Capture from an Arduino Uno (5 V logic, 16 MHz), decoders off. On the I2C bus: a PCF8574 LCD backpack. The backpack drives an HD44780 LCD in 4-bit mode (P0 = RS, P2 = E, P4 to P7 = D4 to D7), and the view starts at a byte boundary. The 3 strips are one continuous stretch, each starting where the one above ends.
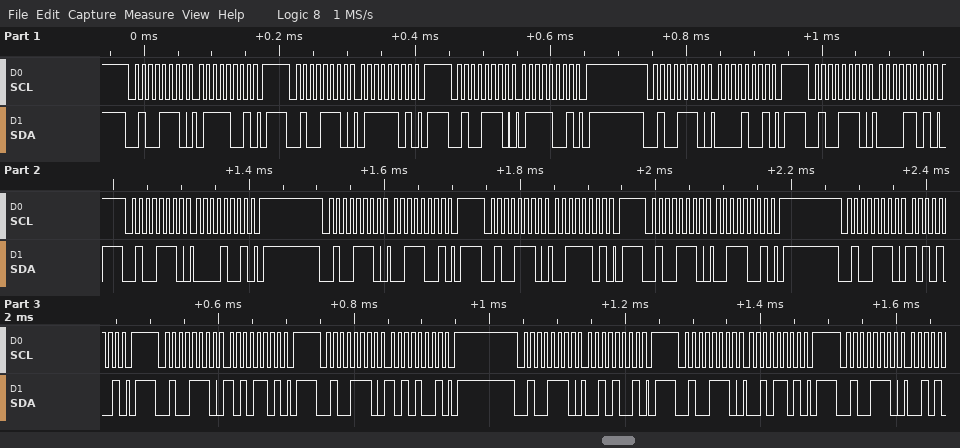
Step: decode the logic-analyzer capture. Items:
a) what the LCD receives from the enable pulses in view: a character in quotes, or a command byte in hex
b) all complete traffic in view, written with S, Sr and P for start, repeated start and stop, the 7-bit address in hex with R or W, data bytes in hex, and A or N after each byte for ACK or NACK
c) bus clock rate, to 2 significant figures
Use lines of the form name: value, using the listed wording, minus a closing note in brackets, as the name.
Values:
what the LCD receives from the enable pulses in view: a character in quotes, or a command byte in hex: 'p' ':'
all complete traffic in view, written with S, Sr and P for start, repeated start and stop, the 7-bit address in hex with R or W, data bytes in hex, and A or N after each byte for ACK or NACK: S 27W A 79 A P S 27W A 7D A P S 27W A 79 A P S 27W A 09 A P S 27W A 0D A P S 27W A 09 A P S 27W A 39 A P S 27W A 3D A P S 27W A 39 A P S 27W A A9 A P S 27W A AD A P S 27W A A9 A P S 27W A 29 A P S 27W A 2D A P S 27W A
bus clock rate, to 2 significant figures: 100 kHz
